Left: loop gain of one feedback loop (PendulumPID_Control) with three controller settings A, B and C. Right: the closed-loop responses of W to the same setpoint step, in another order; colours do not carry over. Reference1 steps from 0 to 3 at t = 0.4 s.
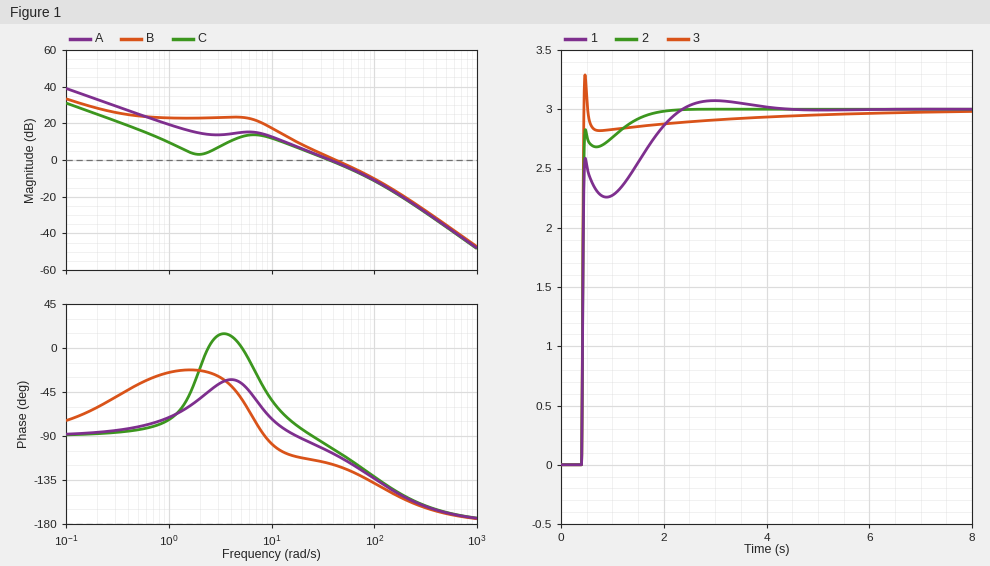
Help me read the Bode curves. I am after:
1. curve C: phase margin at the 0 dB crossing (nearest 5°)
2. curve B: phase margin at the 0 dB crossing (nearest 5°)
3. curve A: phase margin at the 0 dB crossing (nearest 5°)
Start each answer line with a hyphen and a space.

- 80°
- 60°
- 75°
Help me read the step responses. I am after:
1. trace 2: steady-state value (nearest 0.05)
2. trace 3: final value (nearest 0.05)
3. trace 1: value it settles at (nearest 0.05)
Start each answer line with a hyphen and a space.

- 3.00
- 3.00
- 3.00
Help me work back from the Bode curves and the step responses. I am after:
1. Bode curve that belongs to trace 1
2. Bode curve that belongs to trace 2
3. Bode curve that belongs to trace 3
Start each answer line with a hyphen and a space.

- C
- A
- B
